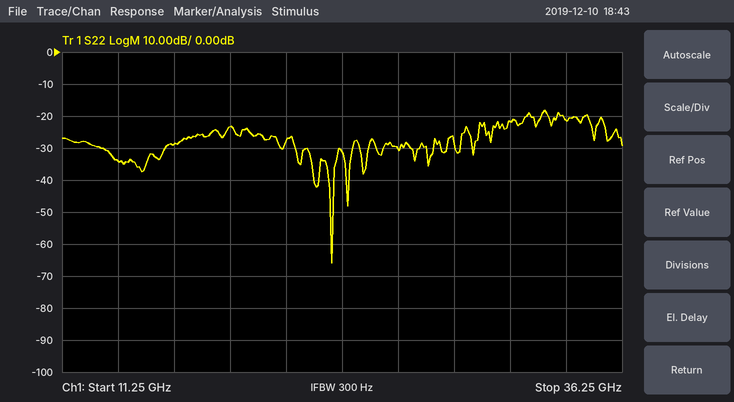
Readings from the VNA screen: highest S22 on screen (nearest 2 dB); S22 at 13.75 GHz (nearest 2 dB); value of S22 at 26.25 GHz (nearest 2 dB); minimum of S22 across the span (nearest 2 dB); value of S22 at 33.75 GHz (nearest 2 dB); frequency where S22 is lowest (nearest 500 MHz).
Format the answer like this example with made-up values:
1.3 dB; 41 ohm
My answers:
-18 dB; -34 dB; -30 dB; -66 dB; -22 dB; 23.5 GHz
